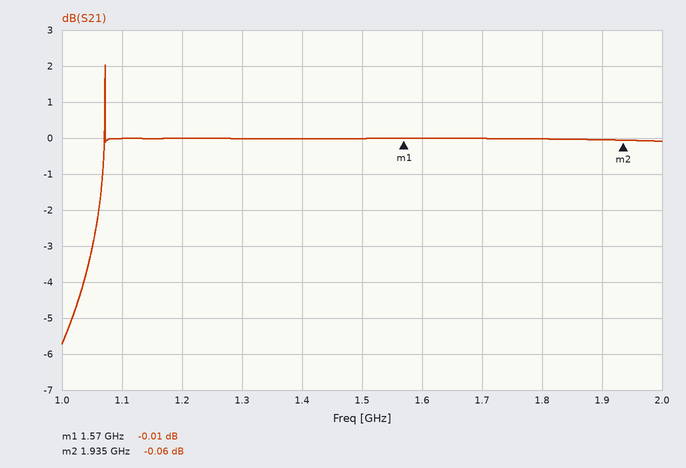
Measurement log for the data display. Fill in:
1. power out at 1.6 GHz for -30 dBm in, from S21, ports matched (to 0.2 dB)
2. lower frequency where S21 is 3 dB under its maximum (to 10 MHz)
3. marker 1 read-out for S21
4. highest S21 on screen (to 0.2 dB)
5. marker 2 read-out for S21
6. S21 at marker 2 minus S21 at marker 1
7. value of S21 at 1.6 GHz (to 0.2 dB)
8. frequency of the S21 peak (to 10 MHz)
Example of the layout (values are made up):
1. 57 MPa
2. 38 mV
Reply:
1. -30.0 dBm
2. 1.07 GHz
3. -0.01 dB
4. 2.0 dB
5. -0.06 dB
6. -0.05 dB
7. 0.0 dB
8. 1.07 GHz
